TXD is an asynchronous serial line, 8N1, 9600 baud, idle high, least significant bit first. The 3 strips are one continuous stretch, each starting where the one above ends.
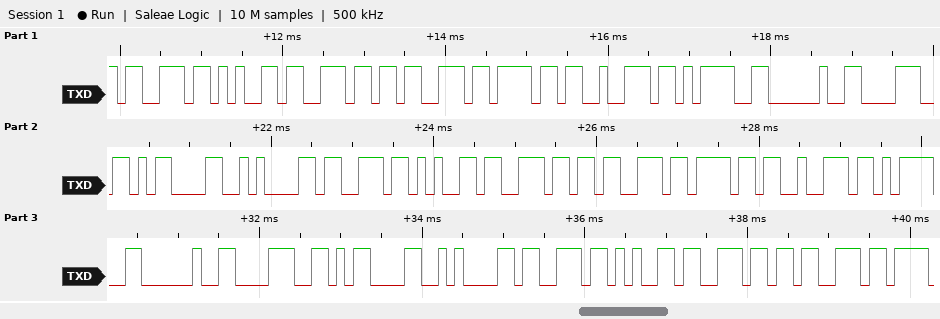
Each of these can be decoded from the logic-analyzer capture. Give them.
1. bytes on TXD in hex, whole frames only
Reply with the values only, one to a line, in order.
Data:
73 65 6E 73 6F 72 3D 20 38 0D 0A 73 65 6E 73 6F 72 3D 20 38 0D 0A 73 65 6E 73
